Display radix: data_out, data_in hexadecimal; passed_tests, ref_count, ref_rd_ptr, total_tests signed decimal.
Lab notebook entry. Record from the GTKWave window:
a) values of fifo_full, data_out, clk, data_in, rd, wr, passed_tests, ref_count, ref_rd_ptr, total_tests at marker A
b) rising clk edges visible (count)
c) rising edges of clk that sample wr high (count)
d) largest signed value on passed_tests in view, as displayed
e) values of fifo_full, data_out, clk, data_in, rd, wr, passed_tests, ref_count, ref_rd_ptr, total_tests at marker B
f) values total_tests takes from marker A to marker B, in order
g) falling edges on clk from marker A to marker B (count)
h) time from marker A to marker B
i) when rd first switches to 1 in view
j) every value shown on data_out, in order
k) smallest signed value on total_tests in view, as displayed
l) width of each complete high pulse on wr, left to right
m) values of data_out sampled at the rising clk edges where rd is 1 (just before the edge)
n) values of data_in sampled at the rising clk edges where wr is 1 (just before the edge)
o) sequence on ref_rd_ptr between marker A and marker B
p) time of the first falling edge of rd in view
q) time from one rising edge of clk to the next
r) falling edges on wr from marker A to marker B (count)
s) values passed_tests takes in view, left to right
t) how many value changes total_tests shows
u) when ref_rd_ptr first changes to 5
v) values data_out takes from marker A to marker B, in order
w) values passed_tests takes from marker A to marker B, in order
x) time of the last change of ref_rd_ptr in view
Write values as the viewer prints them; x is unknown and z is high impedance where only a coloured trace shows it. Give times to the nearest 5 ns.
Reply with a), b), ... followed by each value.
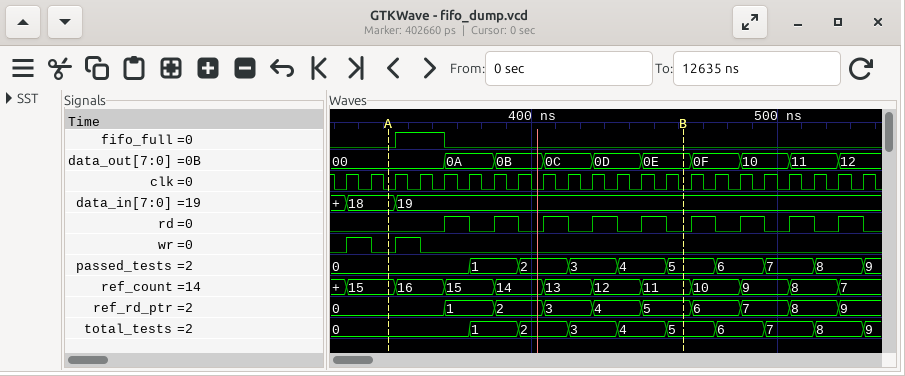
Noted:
a) fifo_full=0, data_out=00, clk=0, data_in=18, rd=0, wr=0, passed_tests=0, ref_count=15, ref_rd_ptr=0, total_tests=0
b) 22
c) 2
d) 9
e) fifo_full=0, data_out=0E, clk=0, data_in=19, rd=0, wr=0, passed_tests=5, ref_count=11, ref_rd_ptr=5, total_tests=5
f) 0, 1, 2, 3, 4, 5
g) 12
h) 120 ns
i) 365 ns
j) 00, 0A, 0B, 0C, 0D, 0E, 0F, 10, 11, 12
k) 0
l) 10 ns, 10 ns
m) 0A, 0B, 0C, 0D, 0E, 0F, 10, 11, 12
n) 18, 19
o) 0, 1, 2, 3, 4, 5
p) 375 ns
q) 10 ns
r) 1
s) 0, 1, 2, 3, 4, 5, 6, 7, 8, 9
t) 9
u) 445 ns
v) 00, 0A, 0B, 0C, 0D, 0E
w) 0, 1, 2, 3, 4, 5
x) 525 ns
